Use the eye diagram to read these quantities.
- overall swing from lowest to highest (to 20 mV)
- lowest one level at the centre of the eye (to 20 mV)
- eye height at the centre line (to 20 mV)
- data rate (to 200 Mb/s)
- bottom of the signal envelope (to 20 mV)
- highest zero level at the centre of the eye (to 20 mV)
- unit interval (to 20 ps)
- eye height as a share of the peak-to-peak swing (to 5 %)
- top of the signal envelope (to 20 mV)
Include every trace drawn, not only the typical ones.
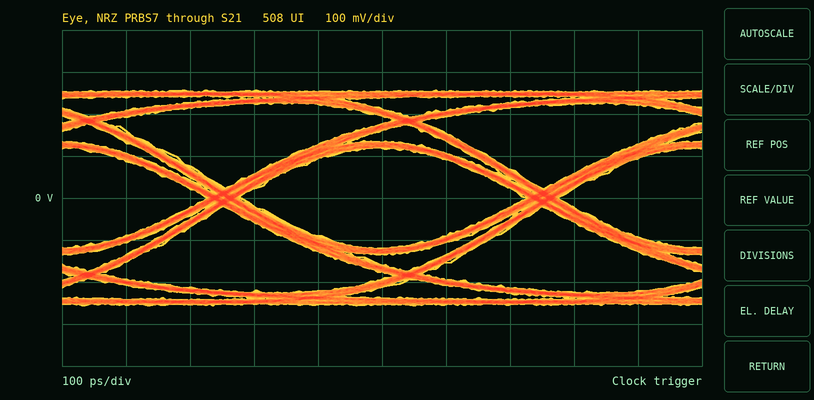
520 mV
120 mV
240 mV
2.0 Gb/s
-260 mV
-120 mV
500 ps
45 %
260 mV
